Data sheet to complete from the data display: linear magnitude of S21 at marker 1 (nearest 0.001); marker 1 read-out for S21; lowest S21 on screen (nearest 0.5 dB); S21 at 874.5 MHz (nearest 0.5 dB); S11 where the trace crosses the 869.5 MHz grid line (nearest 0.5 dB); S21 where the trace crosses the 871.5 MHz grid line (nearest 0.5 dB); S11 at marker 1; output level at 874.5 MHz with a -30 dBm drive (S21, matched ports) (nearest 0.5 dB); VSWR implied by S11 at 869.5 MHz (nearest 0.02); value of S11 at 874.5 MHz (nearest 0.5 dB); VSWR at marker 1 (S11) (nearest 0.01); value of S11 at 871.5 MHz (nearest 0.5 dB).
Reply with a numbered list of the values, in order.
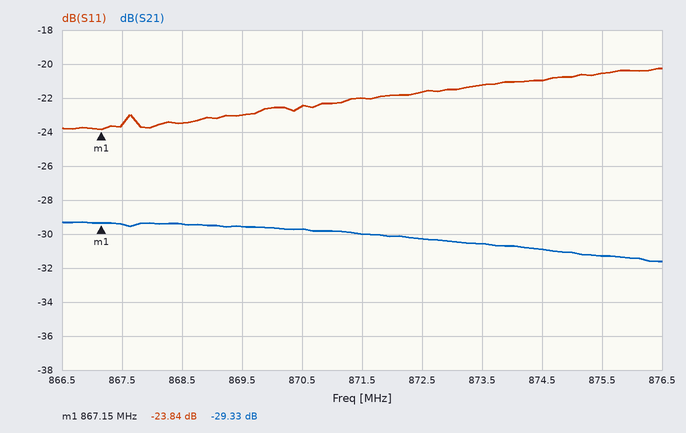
1. 0.034
2. -29.33 dB
3. -31.5 dB
4. -31.0 dB
5. -23.0 dB
6. -30.0 dB
7. -23.84 dB
8. -61.0 dBm
9. 1.16
10. -21.0 dB
11. 1.14
12. -22.0 dB
